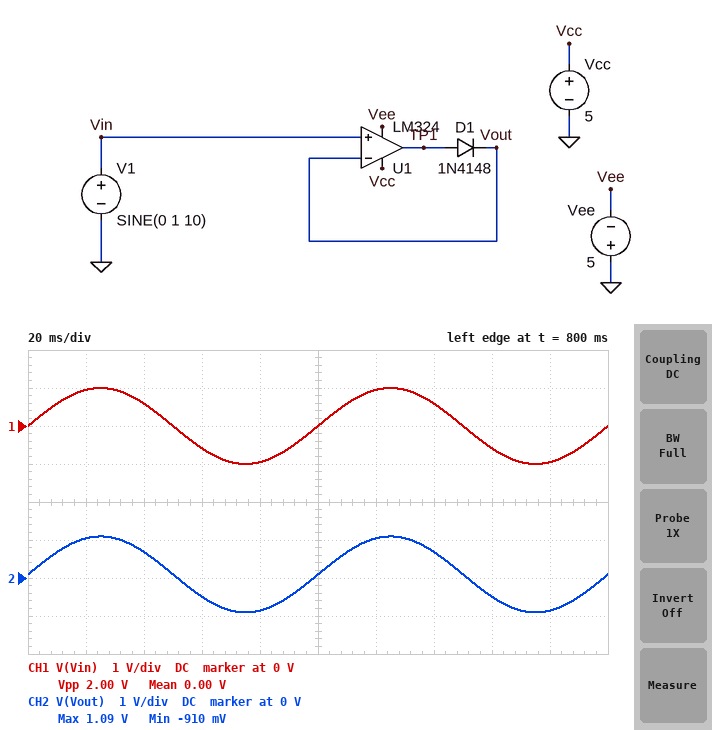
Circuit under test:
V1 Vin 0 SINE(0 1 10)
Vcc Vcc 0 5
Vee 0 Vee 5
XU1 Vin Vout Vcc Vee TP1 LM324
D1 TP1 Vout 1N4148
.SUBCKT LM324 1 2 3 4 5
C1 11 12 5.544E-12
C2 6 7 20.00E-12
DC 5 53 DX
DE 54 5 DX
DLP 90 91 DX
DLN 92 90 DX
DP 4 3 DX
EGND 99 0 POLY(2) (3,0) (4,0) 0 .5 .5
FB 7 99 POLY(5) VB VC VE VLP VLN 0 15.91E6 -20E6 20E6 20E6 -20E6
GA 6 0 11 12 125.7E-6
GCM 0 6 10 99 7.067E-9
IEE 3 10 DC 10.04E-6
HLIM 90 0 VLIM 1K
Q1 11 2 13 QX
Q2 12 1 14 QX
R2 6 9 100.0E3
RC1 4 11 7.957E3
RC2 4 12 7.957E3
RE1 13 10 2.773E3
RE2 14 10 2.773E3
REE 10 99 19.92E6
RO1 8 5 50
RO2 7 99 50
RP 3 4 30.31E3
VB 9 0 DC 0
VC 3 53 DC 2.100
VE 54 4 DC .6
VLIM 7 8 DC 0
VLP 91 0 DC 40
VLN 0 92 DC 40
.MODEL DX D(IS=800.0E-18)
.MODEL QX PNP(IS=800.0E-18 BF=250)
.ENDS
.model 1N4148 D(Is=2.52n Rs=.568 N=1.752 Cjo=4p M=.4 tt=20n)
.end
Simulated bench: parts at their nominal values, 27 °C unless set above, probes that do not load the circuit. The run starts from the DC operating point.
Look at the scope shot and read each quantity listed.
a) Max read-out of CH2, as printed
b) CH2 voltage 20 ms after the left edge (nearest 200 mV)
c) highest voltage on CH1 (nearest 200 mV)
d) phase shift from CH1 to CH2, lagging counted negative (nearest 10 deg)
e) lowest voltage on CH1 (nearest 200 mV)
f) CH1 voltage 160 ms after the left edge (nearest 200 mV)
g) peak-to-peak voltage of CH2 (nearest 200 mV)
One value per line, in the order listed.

1.09 V
1.0 V
1.0 V
0 deg
-1.0 V
-600 mV
2.0 V
